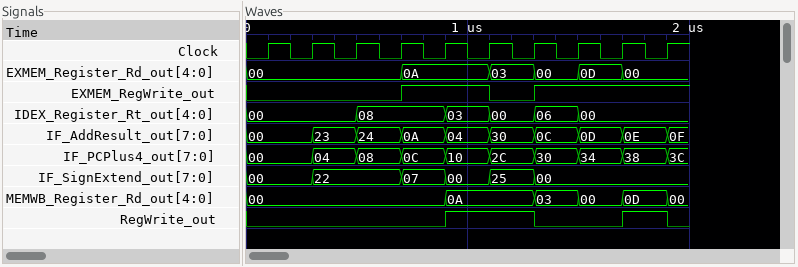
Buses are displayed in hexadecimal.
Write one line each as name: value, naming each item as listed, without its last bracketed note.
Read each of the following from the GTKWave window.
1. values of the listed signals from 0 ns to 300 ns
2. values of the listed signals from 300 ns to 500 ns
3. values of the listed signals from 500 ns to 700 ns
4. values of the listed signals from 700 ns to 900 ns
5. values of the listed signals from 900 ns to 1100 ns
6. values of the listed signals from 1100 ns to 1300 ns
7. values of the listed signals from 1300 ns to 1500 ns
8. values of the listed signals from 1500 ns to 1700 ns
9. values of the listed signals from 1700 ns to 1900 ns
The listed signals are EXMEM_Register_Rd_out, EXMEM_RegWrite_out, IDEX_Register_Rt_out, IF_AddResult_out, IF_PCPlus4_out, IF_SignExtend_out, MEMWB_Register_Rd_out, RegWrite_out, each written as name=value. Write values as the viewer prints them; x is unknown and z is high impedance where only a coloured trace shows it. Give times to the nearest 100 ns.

values of the listed signals from 0 ns to 300 ns: EXMEM_Register_Rd_out=00, EXMEM_RegWrite_out=0, IDEX_Register_Rt_out=00, IF_AddResult_out=00, IF_PCPlus4_out=00, IF_SignExtend_out=00, MEMWB_Register_Rd_out=00, RegWrite_out=0
values of the listed signals from 300 ns to 500 ns: EXMEM_Register_Rd_out=00, EXMEM_RegWrite_out=0, IDEX_Register_Rt_out=00, IF_AddResult_out=23, IF_PCPlus4_out=04, IF_SignExtend_out=22, MEMWB_Register_Rd_out=00, RegWrite_out=0
values of the listed signals from 500 ns to 700 ns: EXMEM_Register_Rd_out=00, EXMEM_RegWrite_out=0, IDEX_Register_Rt_out=08, IF_AddResult_out=24, IF_PCPlus4_out=08, IF_SignExtend_out=22, MEMWB_Register_Rd_out=00, RegWrite_out=0
values of the listed signals from 700 ns to 900 ns: EXMEM_Register_Rd_out=0A, EXMEM_RegWrite_out=1, IDEX_Register_Rt_out=08, IF_AddResult_out=0A, IF_PCPlus4_out=0C, IF_SignExtend_out=07, MEMWB_Register_Rd_out=00, RegWrite_out=0
values of the listed signals from 900 ns to 1100 ns: EXMEM_Register_Rd_out=0A, EXMEM_RegWrite_out=1, IDEX_Register_Rt_out=03, IF_AddResult_out=04, IF_PCPlus4_out=10, IF_SignExtend_out=00, MEMWB_Register_Rd_out=0A, RegWrite_out=1
values of the listed signals from 1100 ns to 1300 ns: EXMEM_Register_Rd_out=03, EXMEM_RegWrite_out=0, IDEX_Register_Rt_out=00, IF_AddResult_out=30, IF_PCPlus4_out=2C, IF_SignExtend_out=25, MEMWB_Register_Rd_out=0A, RegWrite_out=1
values of the listed signals from 1300 ns to 1500 ns: EXMEM_Register_Rd_out=00, EXMEM_RegWrite_out=1, IDEX_Register_Rt_out=06, IF_AddResult_out=0C, IF_PCPlus4_out=30, IF_SignExtend_out=00, MEMWB_Register_Rd_out=03, RegWrite_out=0
values of the listed signals from 1500 ns to 1700 ns: EXMEM_Register_Rd_out=0D, EXMEM_RegWrite_out=1, IDEX_Register_Rt_out=00, IF_AddResult_out=0D, IF_PCPlus4_out=34, IF_SignExtend_out=00, MEMWB_Register_Rd_out=00, RegWrite_out=0
values of the listed signals from 1700 ns to 1900 ns: EXMEM_Register_Rd_out=00, EXMEM_RegWrite_out=1, IDEX_Register_Rt_out=00, IF_AddResult_out=0E, IF_PCPlus4_out=38, IF_SignExtend_out=00, MEMWB_Register_Rd_out=0D, RegWrite_out=1
